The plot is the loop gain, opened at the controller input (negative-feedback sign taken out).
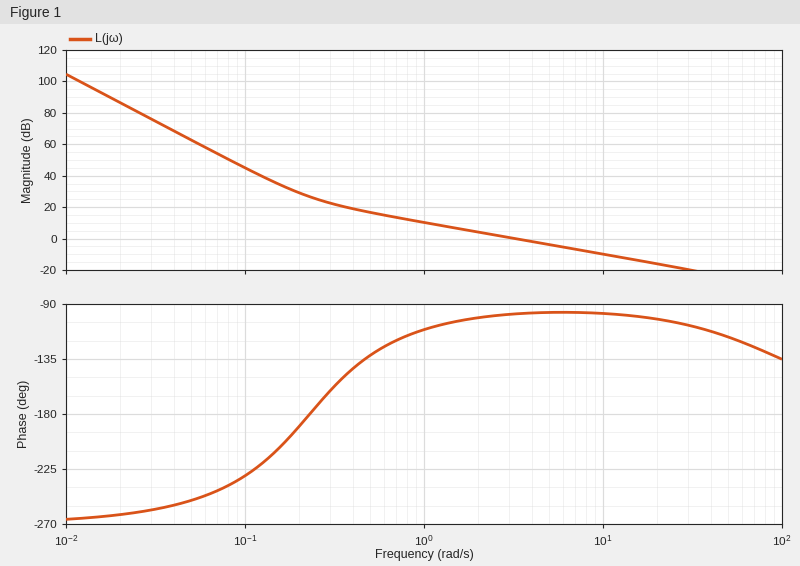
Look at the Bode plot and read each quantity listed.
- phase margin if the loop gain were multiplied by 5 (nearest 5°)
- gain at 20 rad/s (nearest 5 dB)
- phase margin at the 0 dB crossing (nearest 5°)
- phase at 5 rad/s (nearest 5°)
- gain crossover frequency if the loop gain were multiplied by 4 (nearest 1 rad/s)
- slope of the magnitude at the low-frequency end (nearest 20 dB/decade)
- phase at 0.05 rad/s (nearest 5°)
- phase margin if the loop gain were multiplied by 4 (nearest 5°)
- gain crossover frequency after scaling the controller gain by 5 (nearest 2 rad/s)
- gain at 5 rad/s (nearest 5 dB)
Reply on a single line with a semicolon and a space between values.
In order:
80°; -15 dB; 80°; -95°; 13 rad/s; -60 dB/decade; -250°; 80°; 16 rad/s; -5 dB
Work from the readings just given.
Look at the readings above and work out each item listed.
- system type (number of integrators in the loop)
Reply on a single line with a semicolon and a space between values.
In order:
3
